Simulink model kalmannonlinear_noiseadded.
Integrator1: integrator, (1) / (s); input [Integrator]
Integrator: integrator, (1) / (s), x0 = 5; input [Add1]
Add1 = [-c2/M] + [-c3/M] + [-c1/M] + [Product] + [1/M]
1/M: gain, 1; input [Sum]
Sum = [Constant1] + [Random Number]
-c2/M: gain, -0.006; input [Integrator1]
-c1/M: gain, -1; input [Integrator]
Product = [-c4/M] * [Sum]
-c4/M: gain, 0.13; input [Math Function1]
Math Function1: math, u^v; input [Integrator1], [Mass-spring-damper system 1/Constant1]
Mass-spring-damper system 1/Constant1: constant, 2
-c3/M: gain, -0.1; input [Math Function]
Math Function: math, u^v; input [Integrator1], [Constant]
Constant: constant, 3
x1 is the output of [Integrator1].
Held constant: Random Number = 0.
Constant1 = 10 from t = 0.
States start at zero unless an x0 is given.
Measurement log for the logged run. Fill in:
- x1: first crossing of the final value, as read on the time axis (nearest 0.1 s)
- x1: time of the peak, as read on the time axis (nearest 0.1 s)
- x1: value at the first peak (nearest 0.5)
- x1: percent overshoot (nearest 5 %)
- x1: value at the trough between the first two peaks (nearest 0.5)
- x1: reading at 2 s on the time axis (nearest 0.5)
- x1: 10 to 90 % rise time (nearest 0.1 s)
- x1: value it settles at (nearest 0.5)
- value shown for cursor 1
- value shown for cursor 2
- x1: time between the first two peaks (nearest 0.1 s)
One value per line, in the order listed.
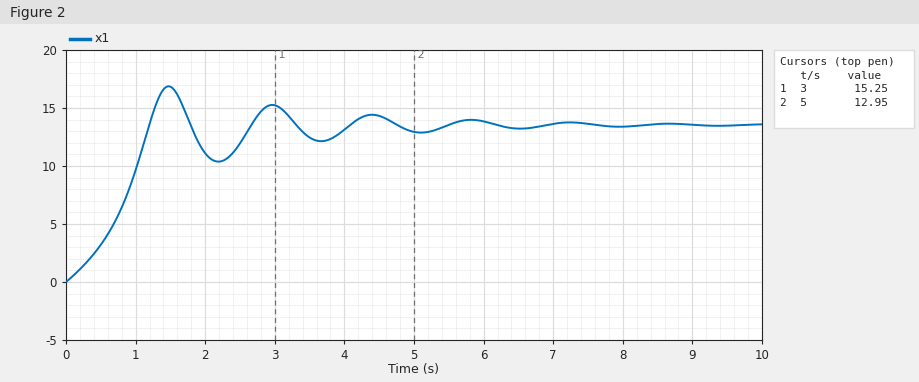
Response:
1.2 s
1.5 s
17.0
25 %
10.5
11.0
0.9 s
13.5
15.25
12.95
1.5 s
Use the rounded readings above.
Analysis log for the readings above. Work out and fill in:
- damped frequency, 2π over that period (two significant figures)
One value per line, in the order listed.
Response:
4.2 rad/s
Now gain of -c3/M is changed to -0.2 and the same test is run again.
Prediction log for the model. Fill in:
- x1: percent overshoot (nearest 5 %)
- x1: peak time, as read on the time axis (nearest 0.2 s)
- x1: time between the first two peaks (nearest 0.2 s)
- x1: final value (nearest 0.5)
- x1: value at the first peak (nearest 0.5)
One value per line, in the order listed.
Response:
25 %
1.2 s
1.8 s
7.5
9.5
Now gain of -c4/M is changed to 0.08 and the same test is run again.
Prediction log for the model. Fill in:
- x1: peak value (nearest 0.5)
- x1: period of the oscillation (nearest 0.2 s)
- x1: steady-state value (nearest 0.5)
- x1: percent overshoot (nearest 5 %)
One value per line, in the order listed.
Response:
11.5
2.0 s
9.0
25 %
